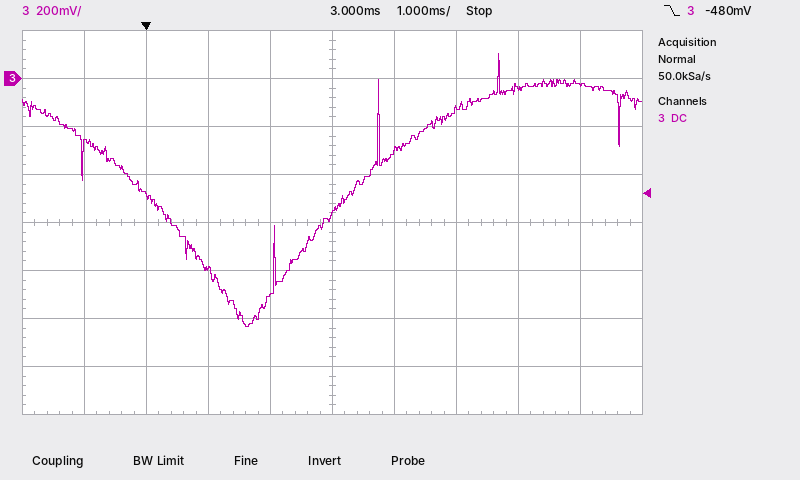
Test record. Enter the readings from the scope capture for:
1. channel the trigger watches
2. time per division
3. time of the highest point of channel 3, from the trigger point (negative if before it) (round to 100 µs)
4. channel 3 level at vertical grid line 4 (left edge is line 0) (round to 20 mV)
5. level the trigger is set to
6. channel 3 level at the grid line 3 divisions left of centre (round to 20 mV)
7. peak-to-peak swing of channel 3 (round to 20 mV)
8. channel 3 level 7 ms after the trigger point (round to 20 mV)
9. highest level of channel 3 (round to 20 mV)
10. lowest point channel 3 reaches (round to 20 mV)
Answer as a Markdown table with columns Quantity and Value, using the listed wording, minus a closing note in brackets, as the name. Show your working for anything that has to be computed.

| Quantity | Value |
|---|---|
| channel the trigger watches | channel 3 |
| time per division | 1 ms |
| time of the highest point of channel 3, from the trigger point (negative if before it) | +5.7 ms |
| channel 3 level at vertical grid line 4 (left edge is line 0) | -900 mV |
| level the trigger is set to | -480 mV |
| channel 3 level at the grid line 3 divisions left of centre | -480 mV |
| peak-to-peak swing of channel 3 | 100 mV − (-1.04 V) = 1.14 V |
| channel 3 level 7 ms after the trigger point | -20 mV |
| highest level of channel 3 | 100 mV |
| lowest point channel 3 reaches | -1.04 V |
